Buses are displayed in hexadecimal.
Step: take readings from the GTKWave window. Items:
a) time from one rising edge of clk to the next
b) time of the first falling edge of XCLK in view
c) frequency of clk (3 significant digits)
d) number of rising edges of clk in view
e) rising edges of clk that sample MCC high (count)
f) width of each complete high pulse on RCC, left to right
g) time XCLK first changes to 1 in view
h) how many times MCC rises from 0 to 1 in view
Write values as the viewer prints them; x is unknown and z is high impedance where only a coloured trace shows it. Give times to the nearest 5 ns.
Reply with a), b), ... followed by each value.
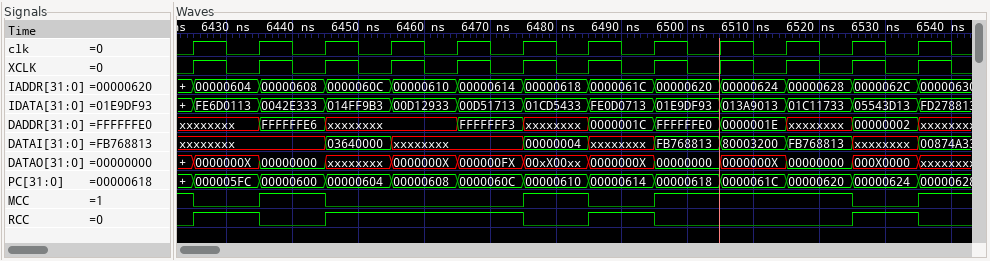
a) 10 ns
b) 6430 ns
c) 100 MHz
d) 12
e) 6
f) 10 ns, 30 ns, 10 ns, 10 ns
g) 6425 ns
h) 4
